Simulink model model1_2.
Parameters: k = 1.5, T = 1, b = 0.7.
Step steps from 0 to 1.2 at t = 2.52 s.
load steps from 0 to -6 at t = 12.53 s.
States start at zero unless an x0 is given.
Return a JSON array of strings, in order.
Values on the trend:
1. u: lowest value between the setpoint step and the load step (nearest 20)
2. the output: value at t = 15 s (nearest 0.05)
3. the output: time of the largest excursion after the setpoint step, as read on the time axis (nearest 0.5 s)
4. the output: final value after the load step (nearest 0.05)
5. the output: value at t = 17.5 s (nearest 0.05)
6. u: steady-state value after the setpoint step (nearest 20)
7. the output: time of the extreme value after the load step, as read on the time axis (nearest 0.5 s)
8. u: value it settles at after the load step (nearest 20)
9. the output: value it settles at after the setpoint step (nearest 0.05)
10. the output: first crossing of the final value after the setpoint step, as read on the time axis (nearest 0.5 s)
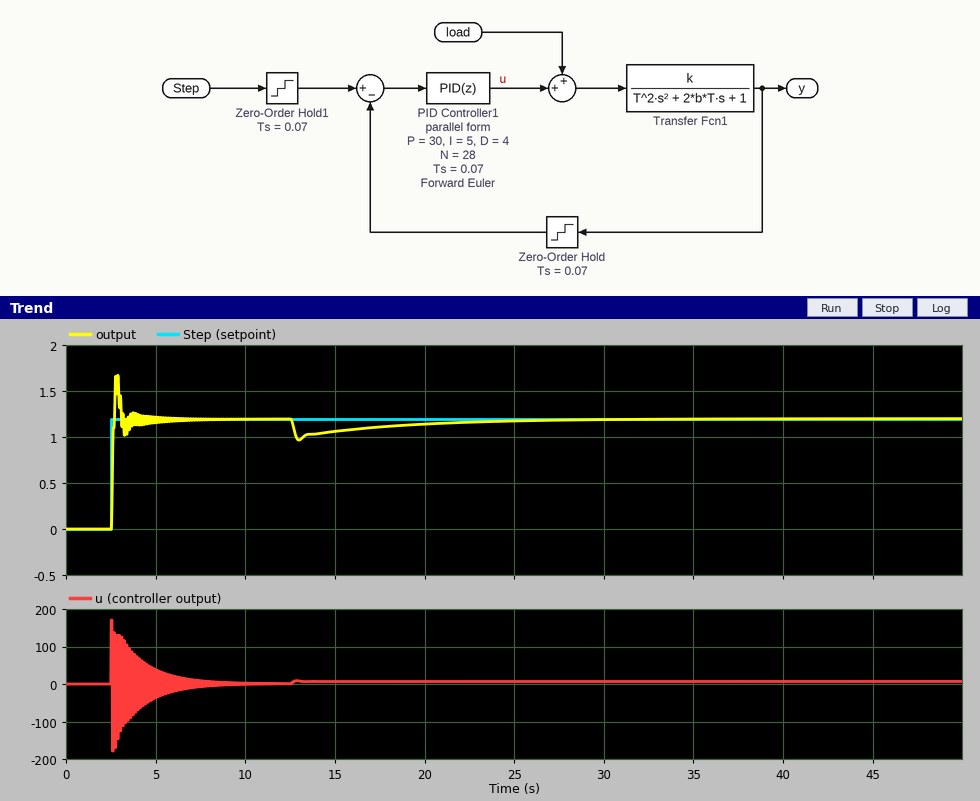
["-180", "1.05", "3.0 s", "1.20", "1.10", "0", "13.0 s", "0", "1.20", "2.5 s"]
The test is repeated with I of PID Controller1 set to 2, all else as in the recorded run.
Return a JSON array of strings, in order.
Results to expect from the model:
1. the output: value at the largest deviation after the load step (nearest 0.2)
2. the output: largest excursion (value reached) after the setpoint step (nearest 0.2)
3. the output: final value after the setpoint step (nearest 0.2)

["1.0", "1.6", "1.2"]
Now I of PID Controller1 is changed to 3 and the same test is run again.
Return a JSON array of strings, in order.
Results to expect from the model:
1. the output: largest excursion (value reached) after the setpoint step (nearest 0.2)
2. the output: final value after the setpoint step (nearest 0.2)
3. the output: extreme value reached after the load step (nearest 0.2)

["1.6", "1.2", "1.0"]
